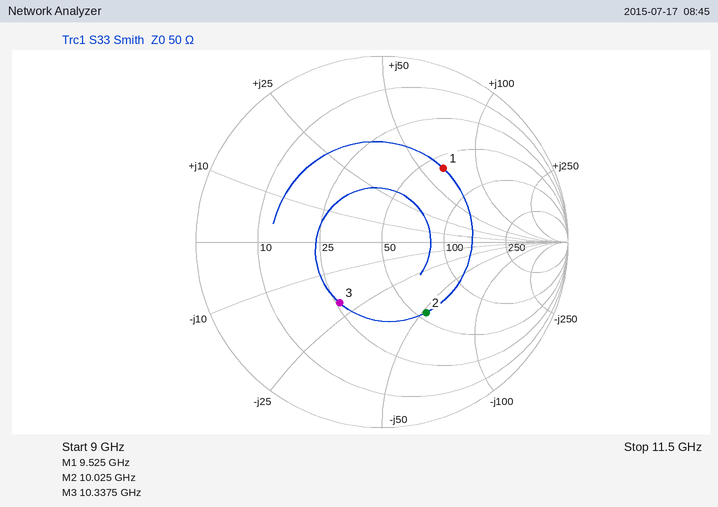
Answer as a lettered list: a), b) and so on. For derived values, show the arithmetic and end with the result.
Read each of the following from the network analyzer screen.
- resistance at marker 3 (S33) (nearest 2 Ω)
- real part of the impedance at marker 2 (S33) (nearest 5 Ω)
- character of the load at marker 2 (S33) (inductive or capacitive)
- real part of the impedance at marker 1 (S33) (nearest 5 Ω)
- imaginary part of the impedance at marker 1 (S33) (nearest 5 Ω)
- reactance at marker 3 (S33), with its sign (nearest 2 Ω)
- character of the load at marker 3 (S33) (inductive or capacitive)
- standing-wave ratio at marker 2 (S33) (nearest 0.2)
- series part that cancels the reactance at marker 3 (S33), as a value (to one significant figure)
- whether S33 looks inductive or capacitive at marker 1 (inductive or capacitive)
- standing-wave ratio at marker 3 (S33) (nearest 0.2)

a) 26 Ω
b) 55 Ω
c) capacitive
d) 60 Ω
e) +65 Ω
f) -20 Ω
g) capacitive
h) 2.6
i) L = 20 Ω/(2π × 10.3375 GHz) ≈ 308 pH, so 300 pH to one significant figure
j) inductive
k) 2.4
